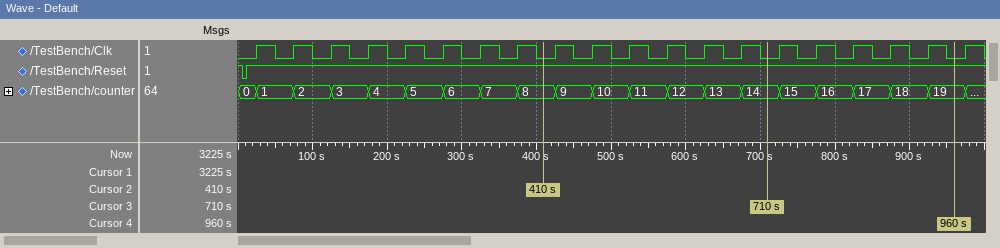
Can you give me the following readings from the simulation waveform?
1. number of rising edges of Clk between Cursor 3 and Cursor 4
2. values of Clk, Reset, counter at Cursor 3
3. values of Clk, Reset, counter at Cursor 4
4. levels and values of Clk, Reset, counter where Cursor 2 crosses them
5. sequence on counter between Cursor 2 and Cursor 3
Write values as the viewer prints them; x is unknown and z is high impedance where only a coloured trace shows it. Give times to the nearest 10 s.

5
Clk=0, Reset=1, counter=14
Clk=0, Reset=1, counter=19
Clk=0, Reset=1, counter=8
8, 9, 10, 11, 12, 13, 14
